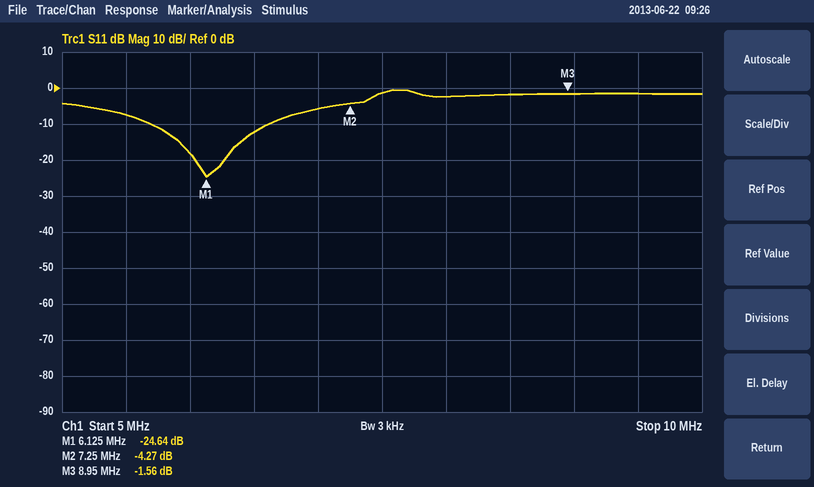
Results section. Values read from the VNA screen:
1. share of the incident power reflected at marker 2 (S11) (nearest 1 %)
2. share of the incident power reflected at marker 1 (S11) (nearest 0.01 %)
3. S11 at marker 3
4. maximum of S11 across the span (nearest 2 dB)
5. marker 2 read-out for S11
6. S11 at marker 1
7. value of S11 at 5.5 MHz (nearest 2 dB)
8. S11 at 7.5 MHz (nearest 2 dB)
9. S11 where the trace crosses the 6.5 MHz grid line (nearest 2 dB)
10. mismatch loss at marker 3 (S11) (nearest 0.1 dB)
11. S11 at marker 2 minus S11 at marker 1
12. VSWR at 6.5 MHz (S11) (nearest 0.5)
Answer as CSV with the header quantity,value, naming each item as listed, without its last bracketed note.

quantity,value
share of the incident power reflected at marker 2 (S11),37 %
share of the incident power reflected at marker 1 (S11),0.34 %
S11 at marker 3,-1.56 dB
maximum of S11 across the span,0 dB
marker 2 read-out for S11,-4.27 dB
S11 at marker 1,-24.64 dB
value of S11 at 5.5 MHz,-8 dB
S11 at 7.5 MHz,-2 dB
S11 where the trace crosses the 6.5 MHz grid line,-12 dB
mismatch loss at marker 3 (S11),5.2 dB
S11 at marker 2 minus S11 at marker 1,20.37 dB
VSWR at 6.5 MHz (S11),1.5
